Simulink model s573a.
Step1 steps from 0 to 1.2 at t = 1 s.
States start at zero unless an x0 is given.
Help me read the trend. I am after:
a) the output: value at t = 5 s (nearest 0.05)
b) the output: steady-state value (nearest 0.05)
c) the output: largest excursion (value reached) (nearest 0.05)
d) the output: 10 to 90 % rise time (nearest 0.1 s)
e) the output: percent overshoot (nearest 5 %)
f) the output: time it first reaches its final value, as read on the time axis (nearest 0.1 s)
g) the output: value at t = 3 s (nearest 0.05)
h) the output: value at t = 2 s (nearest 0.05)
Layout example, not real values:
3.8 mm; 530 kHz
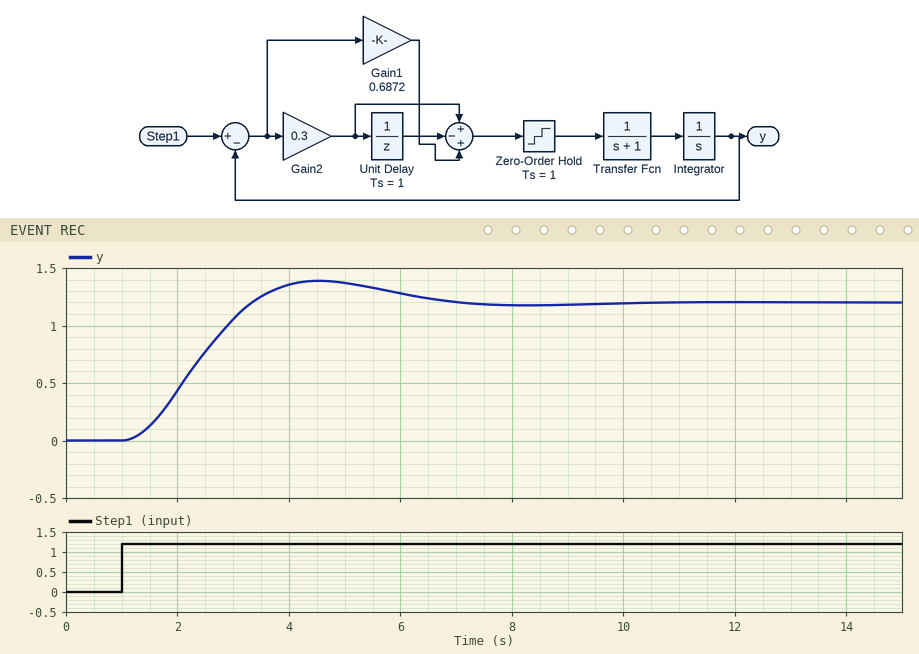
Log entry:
1.35; 1.20; 1.40; 1.6 s; 15 %; 3.3 s; 1.05; 0.45
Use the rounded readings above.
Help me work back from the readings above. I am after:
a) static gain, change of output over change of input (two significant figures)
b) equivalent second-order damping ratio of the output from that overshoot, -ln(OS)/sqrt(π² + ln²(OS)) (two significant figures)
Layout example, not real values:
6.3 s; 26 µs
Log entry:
1.0; 0.52
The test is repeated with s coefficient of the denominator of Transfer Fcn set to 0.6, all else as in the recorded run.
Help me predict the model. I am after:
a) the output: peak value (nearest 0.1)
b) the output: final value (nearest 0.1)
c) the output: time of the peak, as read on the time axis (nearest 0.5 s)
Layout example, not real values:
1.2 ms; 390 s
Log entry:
1.3; 1.2; 3.5 s
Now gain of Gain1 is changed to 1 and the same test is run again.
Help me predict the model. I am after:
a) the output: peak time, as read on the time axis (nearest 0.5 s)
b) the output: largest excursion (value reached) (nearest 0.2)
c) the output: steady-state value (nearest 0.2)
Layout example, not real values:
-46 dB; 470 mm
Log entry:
4.0 s; 1.6; 1.2
